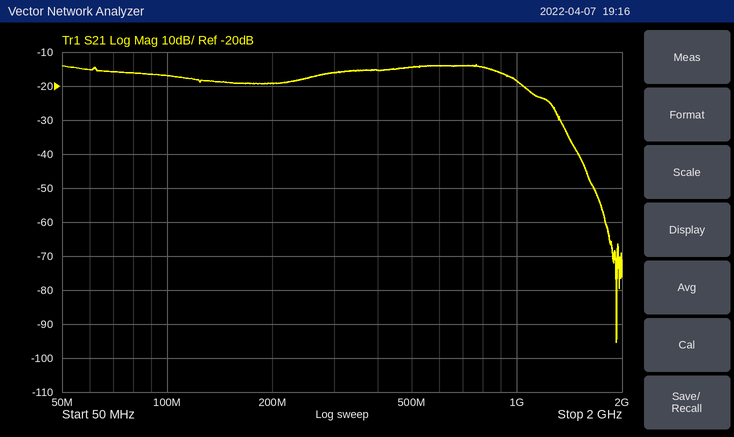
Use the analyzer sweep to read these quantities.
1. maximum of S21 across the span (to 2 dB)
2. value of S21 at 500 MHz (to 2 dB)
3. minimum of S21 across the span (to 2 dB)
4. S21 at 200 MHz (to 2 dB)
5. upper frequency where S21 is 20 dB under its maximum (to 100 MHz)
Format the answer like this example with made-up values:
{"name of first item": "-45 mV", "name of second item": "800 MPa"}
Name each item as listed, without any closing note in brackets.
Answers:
{"maximum of S21 across the span": "-14 dB", "value of S21 at 500 MHz": "-14 dB", "minimum of S21 across the span": "-96 dB", "S21 at 200 MHz": "-20 dB", "upper frequency where S21 is 20 dB under its maximum": "1.4 GHz"}
